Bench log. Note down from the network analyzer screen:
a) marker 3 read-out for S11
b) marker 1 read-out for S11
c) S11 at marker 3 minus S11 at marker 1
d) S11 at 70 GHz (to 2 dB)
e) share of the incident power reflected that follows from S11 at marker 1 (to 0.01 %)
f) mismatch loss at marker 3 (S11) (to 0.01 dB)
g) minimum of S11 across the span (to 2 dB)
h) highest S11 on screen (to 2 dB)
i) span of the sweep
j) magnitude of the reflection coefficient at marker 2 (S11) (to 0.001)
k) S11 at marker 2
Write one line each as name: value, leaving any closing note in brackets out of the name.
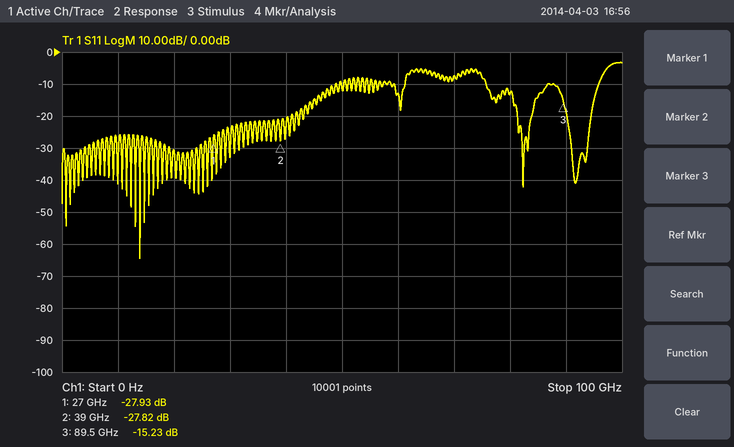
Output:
marker 3 read-out for S11: -15.23 dB
marker 1 read-out for S11: -27.93 dB
S11 at marker 3 minus S11 at marker 1: 12.70 dB
S11 at 70 GHz: -8 dB
share of the incident power reflected that follows from S11 at marker 1: 0.16 %
mismatch loss at marker 3 (S11): 0.13 dB
minimum of S11 across the span: -64 dB
highest S11 on screen: -4 dB
span of the sweep: 100 GHz
magnitude of the reflection coefficient at marker 2 (S11): 0.041
S11 at marker 2: -27.82 dB
